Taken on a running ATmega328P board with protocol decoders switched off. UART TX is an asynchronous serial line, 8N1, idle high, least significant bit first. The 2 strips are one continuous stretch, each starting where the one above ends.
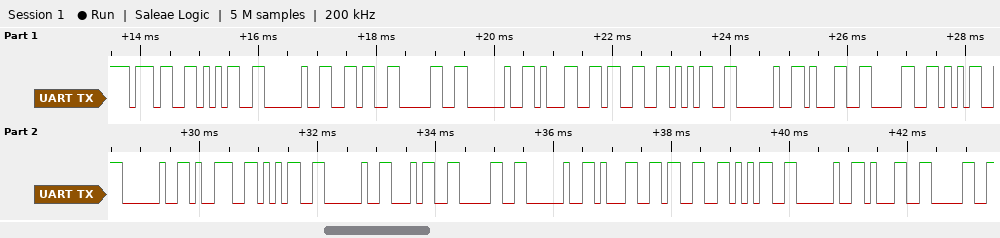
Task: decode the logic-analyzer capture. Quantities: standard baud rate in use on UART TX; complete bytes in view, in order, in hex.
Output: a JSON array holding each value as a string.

["9600 baud", "37 35 20 36 30 20 31 33 35 20 31 30 35 20 39 35 20 34 30 20 31 33 35 20 31 30"]
